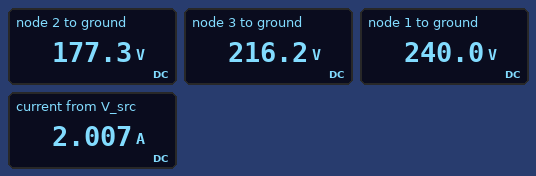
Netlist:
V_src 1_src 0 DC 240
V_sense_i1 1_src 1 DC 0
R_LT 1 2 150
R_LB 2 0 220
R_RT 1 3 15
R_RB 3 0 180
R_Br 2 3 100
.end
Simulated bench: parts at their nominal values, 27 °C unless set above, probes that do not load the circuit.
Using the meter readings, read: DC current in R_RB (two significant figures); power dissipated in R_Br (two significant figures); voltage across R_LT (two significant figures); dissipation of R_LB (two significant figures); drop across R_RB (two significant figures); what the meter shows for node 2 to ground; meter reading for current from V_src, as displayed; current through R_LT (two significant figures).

1.2 A
15 W
63 V
140 W
220 V
177.3 V
2.007 A
420 mA
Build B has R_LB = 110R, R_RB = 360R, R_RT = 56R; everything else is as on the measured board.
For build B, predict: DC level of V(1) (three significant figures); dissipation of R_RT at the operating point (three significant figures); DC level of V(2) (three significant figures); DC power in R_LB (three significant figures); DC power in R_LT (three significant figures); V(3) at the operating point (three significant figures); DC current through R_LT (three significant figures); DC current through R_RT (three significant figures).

240 V
57.2 W
133 V
162 W
75.9 W
183 V
711 mA
1.01 A
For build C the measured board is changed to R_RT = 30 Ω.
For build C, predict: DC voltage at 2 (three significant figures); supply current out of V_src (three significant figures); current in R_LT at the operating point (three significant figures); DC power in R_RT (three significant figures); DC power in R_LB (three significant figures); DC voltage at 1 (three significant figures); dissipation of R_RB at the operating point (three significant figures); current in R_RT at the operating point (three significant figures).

169 V
1.87 A
474 mA
58.3 W
130 W
240 V
218 W
1.39 A
